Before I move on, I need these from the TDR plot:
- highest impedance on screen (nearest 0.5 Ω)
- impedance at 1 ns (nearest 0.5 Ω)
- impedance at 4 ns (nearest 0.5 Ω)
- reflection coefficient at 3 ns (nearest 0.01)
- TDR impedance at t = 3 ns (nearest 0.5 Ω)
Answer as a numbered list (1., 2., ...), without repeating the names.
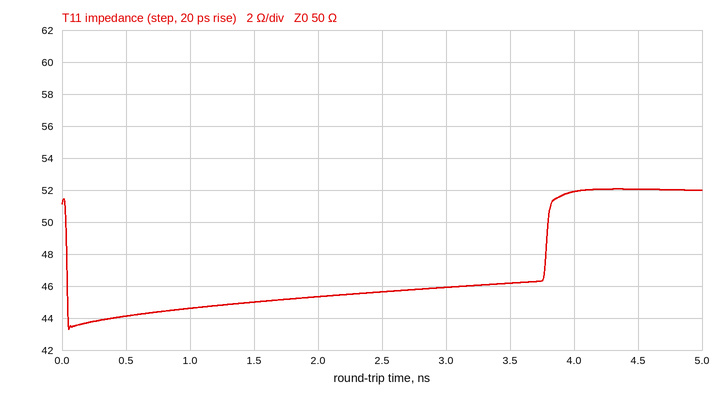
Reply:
1. 52.0 Ω
2. 44.5 Ω
3. 52.0 Ω
4. -0.04
5. 46.0 Ω
